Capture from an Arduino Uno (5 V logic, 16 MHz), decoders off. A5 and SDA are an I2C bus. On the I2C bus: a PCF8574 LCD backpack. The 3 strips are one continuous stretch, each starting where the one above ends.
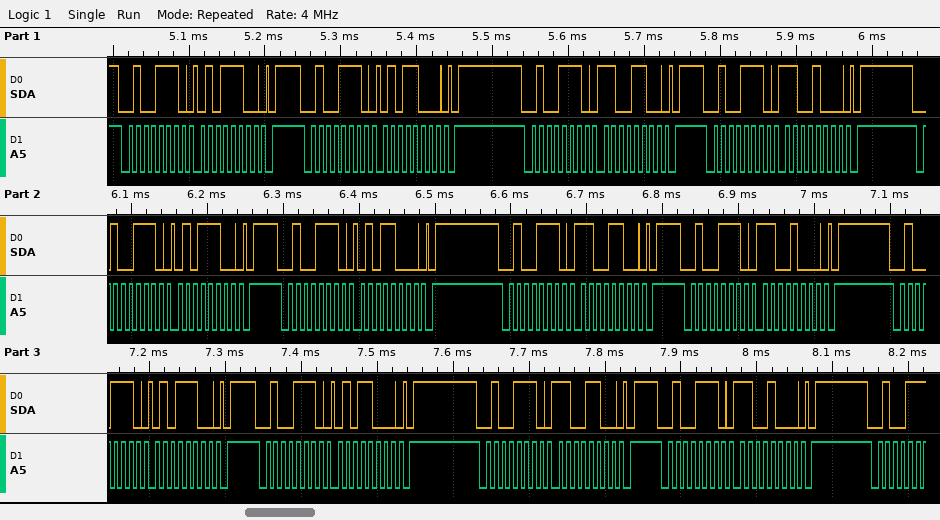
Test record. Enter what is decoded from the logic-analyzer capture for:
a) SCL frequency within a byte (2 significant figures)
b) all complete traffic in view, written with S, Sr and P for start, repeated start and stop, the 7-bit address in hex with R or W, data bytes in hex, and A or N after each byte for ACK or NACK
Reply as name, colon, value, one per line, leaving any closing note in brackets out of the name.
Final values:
SCL frequency within a byte: 100 kHz
all complete traffic in view, written with S, Sr and P for start, repeated start and stop, the 7-bit address in hex with R or W, data bytes in hex, and A or N after each byte for ACK or NACK: S 27W A 5C A P S 27W A 58 A P S 27W A CC A P S 27W A C8 A P S 27W A 5C A P S 27W A 58 A P S 27W A CC A P S 27W A C8 A P S 27W A 5C A P S 27W A 58 A P S 27W A CC A P S 27W A C8 A P
